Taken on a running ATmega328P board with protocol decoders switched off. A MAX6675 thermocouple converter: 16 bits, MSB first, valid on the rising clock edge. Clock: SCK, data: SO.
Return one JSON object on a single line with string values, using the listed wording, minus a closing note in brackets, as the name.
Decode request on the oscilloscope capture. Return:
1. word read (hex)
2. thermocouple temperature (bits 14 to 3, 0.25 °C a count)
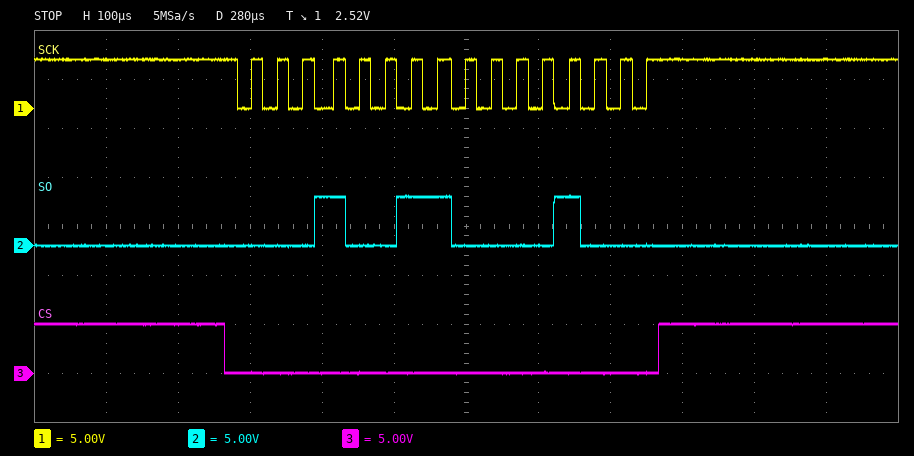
{"word read": "0x1308", "thermocouple temperature": "152.25 °C"}
